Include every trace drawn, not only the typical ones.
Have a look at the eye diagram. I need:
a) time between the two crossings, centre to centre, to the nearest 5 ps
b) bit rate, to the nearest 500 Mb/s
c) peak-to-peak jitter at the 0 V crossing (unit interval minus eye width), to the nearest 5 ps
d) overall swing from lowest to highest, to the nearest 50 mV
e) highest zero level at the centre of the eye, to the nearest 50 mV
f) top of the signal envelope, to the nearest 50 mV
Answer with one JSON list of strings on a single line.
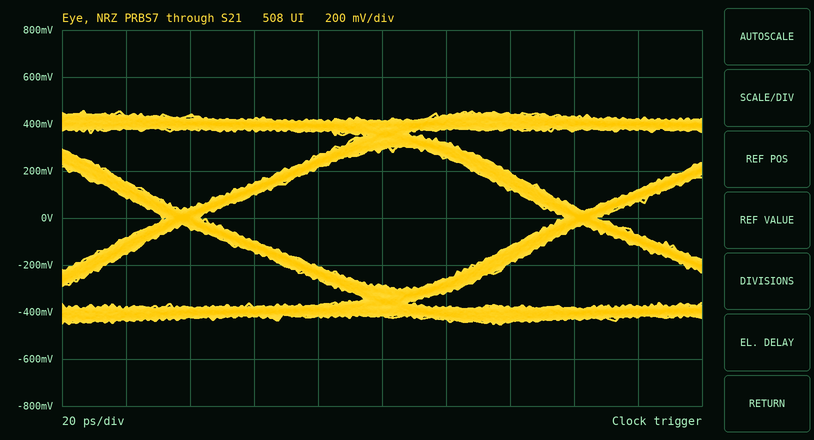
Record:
["125 ps", "8.0 Gb/s", "10 ps", "900 mV", "-300 mV", "450 mV"]
